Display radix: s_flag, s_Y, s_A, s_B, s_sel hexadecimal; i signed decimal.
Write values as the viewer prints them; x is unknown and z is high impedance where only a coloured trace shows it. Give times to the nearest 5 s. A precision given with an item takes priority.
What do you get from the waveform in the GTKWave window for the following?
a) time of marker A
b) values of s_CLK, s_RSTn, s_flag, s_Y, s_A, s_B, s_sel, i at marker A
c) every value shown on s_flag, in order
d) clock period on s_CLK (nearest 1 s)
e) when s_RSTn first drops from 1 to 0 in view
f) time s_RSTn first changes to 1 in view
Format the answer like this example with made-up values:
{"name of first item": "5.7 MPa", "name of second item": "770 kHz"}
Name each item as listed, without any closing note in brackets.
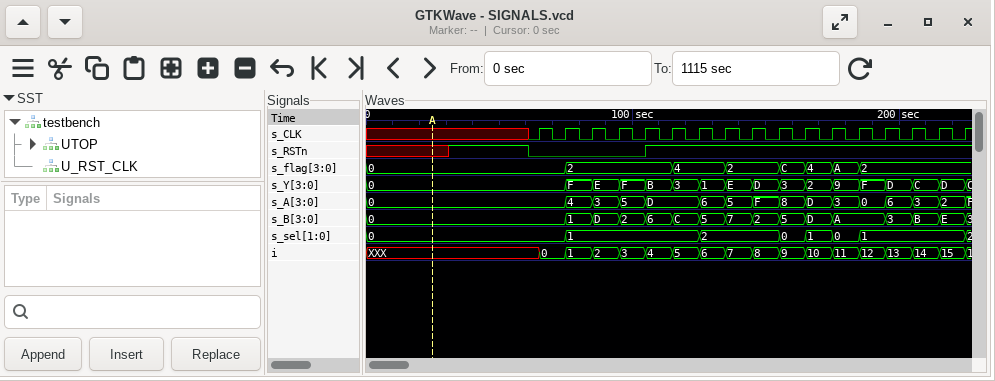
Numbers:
{"time of marker A": "25 s", "values of s_CLK, s_RSTn, s_flag, s_Y, s_A, s_B, s_sel, i at marker A": "s_CLK=x, s_RSTn=x, s_flag=0, s_Y=0, s_A=0, s_B=0, s_sel=0, i=XXX", "every value shown on s_flag, in order": "0, 2, 4, 2, C, 4, A, 2", "clock period on s_CLK": "10 s", "when s_RSTn first drops from 1 to 0 in view": "60 s", "time s_RSTn first changes to 1 in view": "30 s"}
